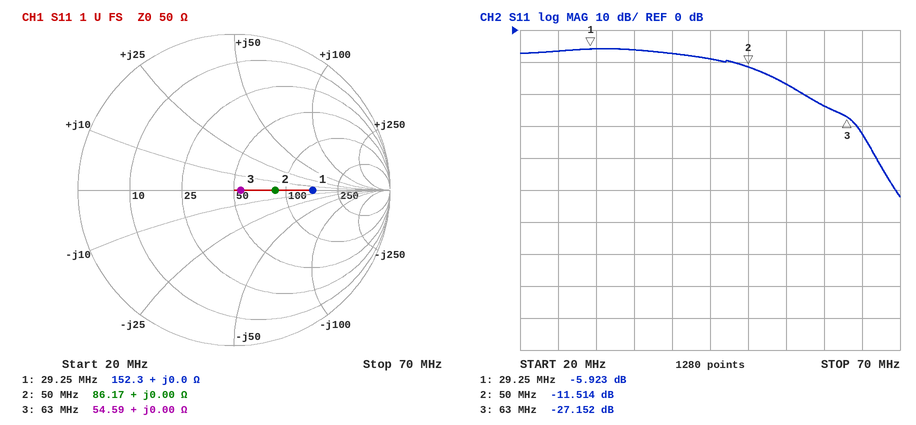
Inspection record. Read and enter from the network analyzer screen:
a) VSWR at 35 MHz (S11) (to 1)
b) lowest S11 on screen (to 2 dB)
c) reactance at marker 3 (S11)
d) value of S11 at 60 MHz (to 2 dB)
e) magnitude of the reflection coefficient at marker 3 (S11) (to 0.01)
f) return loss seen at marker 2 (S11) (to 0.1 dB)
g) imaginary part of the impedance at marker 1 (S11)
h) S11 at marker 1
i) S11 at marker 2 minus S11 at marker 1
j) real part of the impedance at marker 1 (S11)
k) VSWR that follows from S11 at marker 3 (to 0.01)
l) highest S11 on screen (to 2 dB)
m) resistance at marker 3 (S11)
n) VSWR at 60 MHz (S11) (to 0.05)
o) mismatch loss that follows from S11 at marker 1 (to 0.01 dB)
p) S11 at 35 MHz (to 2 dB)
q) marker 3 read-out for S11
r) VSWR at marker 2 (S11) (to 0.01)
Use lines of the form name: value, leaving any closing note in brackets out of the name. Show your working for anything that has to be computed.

VSWR at 35 MHz (S11): |Γ| = 10^(-6/20) = 0.5012; VSWR = (1 + 0.5012)/(1 − 0.5012) ≈ 3
lowest S11 on screen: -52 dB
reactance at marker 3: +0.00 Ω
value of S11 at 60 MHz: -24 dB
magnitude of the reflection coefficient at marker 3 (S11): 0.04
return loss seen at marker 2 (S11): 11.5 dB
imaginary part of the impedance at marker 1: +0.0 Ω
S11 at marker 1: -5.923 dB
S11 at marker 2 minus S11 at marker 1: -11.514 − (-5.923) = -5.591 dB
real part of the impedance at marker 1: 152.3 Ω
VSWR that follows from S11 at marker 3: (1 + 0.0439)/(1 − 0.0439) ≈ 1.09
highest S11 on screen: -6 dB
resistance at marker 3: 54.59 Ω
VSWR at 60 MHz (S11): |Γ| = 10^(-24/20) = 0.0631; VSWR = (1 + 0.0631)/(1 − 0.0631) ≈ 1.13, so 1.15 to the nearest 0.05
mismatch loss that follows from S11 at marker 1: −10 log10(1 − 10^(-5.923/10)) ≈ 1.28 dB
S11 at 35 MHz: -6 dB
marker 3 read-out for S11: -27.152 dB
VSWR at marker 2 (S11): (1 + 0.2656)/(1 − 0.2656) ≈ 1.72
